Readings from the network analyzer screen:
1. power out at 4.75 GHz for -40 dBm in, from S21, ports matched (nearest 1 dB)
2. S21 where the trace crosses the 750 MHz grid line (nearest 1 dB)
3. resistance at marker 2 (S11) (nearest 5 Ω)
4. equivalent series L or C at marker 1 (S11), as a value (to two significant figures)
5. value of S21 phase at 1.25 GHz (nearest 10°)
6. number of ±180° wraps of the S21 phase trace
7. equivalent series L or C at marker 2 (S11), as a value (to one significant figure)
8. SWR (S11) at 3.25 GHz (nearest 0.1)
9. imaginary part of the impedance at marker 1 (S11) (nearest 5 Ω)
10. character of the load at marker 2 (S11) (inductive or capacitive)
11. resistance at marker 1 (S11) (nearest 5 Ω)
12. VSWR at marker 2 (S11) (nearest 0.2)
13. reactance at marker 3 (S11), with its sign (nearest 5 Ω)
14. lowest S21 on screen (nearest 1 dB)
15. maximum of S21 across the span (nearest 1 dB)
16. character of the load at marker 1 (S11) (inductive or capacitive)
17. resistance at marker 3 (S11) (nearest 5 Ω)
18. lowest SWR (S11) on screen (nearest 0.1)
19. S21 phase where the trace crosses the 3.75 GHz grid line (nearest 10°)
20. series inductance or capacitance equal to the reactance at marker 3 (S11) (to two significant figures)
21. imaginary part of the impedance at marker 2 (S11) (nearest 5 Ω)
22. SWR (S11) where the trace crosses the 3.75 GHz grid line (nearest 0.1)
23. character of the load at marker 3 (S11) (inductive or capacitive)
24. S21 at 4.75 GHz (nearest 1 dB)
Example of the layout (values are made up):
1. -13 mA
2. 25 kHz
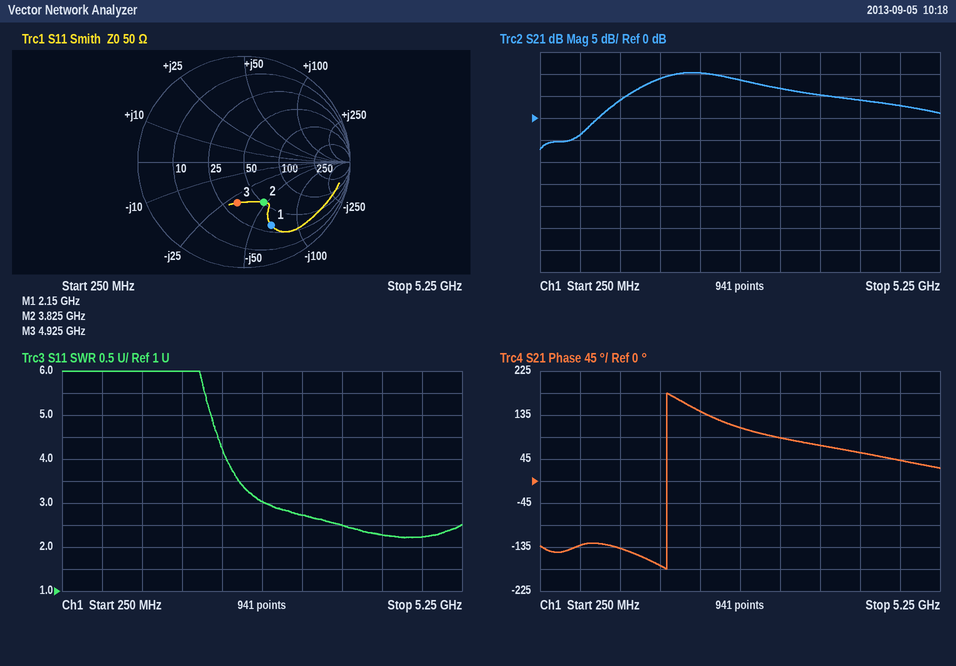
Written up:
1. -37 dBm
2. -4 dB
3. 50 Ω
4. 1.1 pF
5. -140°
6. 1
7. 900 fF
8. 2.7
9. -65 Ω
10. capacitive
11. 30 Ω
12. 2.4
13. -30 Ω
14. -7 dB
15. 10 dB
16. capacitive
17. 35 Ω
18. 2.2
19. 70°
20. 1.1 pF
21. -45 Ω
22. 2.5
23. capacitive
24. 3 dB
